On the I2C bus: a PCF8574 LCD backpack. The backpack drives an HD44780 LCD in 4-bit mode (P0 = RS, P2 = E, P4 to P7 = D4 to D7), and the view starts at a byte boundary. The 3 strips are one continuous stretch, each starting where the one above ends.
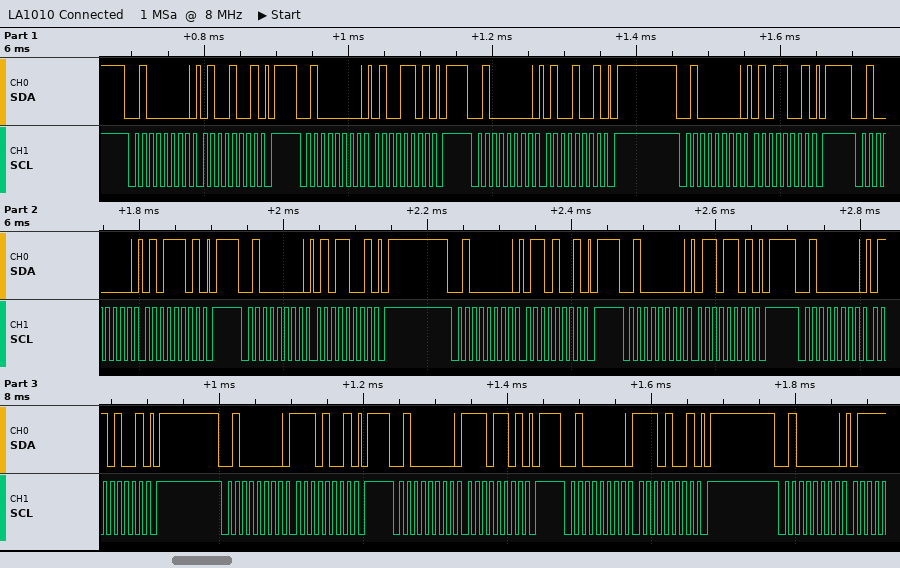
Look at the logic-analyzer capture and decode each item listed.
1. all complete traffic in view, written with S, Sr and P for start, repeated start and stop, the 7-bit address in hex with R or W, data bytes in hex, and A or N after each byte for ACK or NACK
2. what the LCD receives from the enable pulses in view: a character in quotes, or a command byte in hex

S 20W A 49 A P S 20W A 4D A P S 20W A 49 A P S 20W A 59 A P S 20W A 5D A P S 20W A 59 A P S 20W A 69 A P S 20W A 6D A P S 20W A 69 A P S 20W A E9 A P S 20W A ED A P S 20W A E9 A P S 20W A
'E' 'n'
